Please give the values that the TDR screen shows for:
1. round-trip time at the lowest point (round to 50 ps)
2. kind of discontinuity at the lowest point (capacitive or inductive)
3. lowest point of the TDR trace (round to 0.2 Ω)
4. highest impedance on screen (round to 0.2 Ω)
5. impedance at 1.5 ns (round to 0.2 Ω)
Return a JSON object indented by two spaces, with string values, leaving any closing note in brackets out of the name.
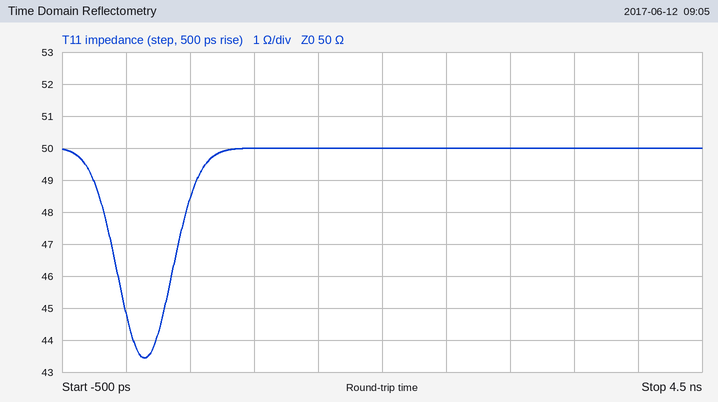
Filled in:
{
  "round-trip time at the lowest point": "150 ps",
  "kind of discontinuity at the lowest point": "capacitive",
  "lowest point of the TDR trace": "43.4 Ω",
  "highest impedance on screen": "50.0 Ω",
  "impedance at 1.5 ns": "50.0 Ω"
}
